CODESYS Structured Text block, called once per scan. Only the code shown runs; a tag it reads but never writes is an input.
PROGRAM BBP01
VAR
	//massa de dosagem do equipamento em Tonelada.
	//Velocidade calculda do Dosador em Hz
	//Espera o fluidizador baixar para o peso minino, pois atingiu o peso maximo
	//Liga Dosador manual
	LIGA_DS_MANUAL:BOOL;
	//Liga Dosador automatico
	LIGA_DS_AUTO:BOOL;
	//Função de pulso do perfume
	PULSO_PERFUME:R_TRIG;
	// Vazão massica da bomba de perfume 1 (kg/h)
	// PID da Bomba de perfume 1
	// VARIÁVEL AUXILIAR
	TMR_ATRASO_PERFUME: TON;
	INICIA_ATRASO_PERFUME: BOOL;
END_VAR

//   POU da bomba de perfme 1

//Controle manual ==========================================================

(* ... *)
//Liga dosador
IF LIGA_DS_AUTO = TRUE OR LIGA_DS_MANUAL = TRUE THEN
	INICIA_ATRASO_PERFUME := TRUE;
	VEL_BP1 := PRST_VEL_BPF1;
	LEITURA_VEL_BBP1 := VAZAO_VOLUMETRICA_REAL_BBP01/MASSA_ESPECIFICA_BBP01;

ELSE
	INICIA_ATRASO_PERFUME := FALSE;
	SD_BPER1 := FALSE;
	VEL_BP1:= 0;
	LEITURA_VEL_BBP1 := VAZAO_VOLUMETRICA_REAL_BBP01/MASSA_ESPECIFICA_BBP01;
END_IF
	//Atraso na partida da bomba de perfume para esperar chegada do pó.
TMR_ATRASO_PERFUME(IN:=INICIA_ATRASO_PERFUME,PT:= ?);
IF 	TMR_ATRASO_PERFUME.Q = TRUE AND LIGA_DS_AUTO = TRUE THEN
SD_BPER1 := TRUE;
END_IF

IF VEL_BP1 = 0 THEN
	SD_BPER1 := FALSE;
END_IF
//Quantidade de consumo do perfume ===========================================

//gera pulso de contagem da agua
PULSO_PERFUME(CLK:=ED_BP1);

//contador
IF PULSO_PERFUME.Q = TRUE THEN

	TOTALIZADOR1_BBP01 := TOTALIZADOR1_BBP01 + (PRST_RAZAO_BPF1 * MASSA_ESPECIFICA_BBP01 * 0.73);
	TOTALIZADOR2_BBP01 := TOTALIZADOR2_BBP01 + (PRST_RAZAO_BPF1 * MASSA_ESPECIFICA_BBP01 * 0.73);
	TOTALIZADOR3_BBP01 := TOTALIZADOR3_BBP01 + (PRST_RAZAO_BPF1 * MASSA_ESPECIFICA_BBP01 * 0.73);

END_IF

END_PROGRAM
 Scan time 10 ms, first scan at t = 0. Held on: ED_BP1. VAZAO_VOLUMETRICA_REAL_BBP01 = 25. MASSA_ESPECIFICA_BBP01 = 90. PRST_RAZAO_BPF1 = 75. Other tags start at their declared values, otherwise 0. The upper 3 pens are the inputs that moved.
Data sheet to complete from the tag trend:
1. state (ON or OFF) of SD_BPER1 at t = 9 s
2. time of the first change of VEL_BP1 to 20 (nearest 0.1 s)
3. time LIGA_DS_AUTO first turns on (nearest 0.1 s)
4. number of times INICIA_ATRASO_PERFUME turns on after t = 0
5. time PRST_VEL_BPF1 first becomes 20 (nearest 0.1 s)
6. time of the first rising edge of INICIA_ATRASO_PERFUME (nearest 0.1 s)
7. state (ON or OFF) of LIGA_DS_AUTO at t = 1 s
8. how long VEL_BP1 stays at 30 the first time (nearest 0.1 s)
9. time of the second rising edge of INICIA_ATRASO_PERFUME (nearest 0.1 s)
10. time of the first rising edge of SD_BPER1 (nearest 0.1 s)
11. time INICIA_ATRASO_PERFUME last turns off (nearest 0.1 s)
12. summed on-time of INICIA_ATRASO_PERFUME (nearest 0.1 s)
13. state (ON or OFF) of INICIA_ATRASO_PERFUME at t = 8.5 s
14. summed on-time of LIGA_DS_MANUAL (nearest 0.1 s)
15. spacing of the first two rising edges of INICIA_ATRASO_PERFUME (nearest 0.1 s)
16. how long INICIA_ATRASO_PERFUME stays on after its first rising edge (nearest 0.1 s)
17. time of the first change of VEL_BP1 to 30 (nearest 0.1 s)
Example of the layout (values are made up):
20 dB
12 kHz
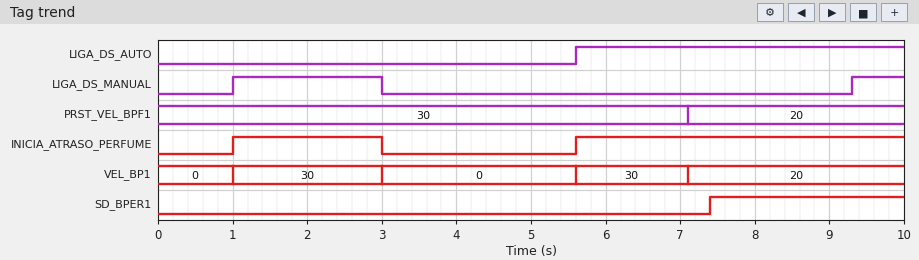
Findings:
ON
7.1 s
5.6 s
2
7.1 s
1.0 s
OFF
2.0 s
5.6 s
7.4 s
3.0 s
6.4 s
ON
2.7 s
4.6 s
2.0 s
1.0 s
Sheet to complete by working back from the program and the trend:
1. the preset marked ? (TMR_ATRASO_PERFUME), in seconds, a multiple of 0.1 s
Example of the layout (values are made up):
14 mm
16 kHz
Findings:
1.8 s
